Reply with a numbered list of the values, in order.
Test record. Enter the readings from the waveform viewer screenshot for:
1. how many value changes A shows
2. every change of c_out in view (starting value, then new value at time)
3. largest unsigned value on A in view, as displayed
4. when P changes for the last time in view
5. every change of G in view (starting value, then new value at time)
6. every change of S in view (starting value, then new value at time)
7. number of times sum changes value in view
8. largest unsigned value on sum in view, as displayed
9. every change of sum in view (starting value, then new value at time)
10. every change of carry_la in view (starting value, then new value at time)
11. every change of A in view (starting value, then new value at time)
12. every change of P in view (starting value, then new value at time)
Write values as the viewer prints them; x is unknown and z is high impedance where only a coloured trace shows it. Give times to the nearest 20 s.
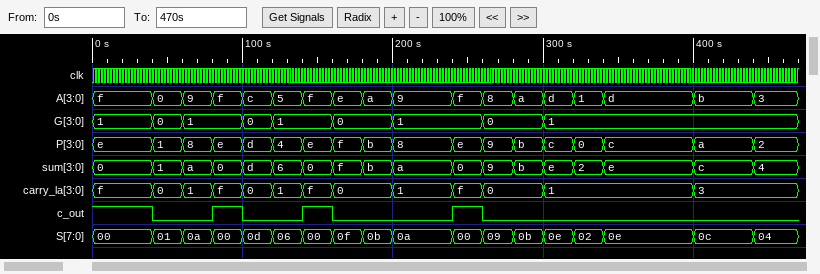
1. 17
2. 1, 0 at 40 s, 1 at 80 s, 0 at 100 s, 1 at 140 s, 0 at 160 s, 1 at 240 s, 0 at 260 s
3. f
4. 440 s
5. 1, 0 at 40 s, 1 at 60 s, 0 at 100 s, 1 at 120 s, 0 at 160 s, 1 at 200 s, 0 at 260 s, 1 at 300 s
6. 00, 01 at 40 s, 0a at 60 s, 00 at 80 s, 0d at 100 s, 06 at 120 s, 00 at 140 s, 0f at 160 s, 0b at 180 s, 0a at 200 s, 00 at 240 s, 09 at 260 s, 0b at 280 s, 0e at 300 s, 02 at 320 s, 0e at 340 s, 0c at 400 s, 04 at 440 s
7. 17
8. f
9. 0, 1 at 40 s, a at 60 s, 0 at 80 s, d at 100 s, 6 at 120 s, 0 at 140 s, f at 160 s, b at 180 s, a at 200 s, 0 at 240 s, 9 at 260 s, b at 280 s, e at 300 s, 2 at 320 s, e at 340 s, c at 400 s, 4 at 440 s
10. f, 0 at 40 s, 1 at 60 s, f at 80 s, 0 at 100 s, 1 at 120 s, f at 140 s, 0 at 160 s, 1 at 200 s, f at 240 s, 0 at 260 s, 1 at 300 s, 3 at 400 s
11. f, 0 at 40 s, 9 at 60 s, f at 80 s, c at 100 s, 5 at 120 s, f at 140 s, e at 160 s, a at 180 s, 9 at 200 s, f at 240 s, 8 at 260 s, a at 280 s, d at 300 s, 1 at 320 s, d at 340 s, b at 400 s, 3 at 440 s
12. e, 1 at 40 s, 8 at 60 s, e at 80 s, d at 100 s, 4 at 120 s, e at 140 s, f at 160 s, b at 180 s, 8 at 200 s, e at 240 s, 9 at 260 s, b at 280 s, c at 300 s, 0 at 320 s, c at 340 s, a at 400 s, 2 at 440 s
